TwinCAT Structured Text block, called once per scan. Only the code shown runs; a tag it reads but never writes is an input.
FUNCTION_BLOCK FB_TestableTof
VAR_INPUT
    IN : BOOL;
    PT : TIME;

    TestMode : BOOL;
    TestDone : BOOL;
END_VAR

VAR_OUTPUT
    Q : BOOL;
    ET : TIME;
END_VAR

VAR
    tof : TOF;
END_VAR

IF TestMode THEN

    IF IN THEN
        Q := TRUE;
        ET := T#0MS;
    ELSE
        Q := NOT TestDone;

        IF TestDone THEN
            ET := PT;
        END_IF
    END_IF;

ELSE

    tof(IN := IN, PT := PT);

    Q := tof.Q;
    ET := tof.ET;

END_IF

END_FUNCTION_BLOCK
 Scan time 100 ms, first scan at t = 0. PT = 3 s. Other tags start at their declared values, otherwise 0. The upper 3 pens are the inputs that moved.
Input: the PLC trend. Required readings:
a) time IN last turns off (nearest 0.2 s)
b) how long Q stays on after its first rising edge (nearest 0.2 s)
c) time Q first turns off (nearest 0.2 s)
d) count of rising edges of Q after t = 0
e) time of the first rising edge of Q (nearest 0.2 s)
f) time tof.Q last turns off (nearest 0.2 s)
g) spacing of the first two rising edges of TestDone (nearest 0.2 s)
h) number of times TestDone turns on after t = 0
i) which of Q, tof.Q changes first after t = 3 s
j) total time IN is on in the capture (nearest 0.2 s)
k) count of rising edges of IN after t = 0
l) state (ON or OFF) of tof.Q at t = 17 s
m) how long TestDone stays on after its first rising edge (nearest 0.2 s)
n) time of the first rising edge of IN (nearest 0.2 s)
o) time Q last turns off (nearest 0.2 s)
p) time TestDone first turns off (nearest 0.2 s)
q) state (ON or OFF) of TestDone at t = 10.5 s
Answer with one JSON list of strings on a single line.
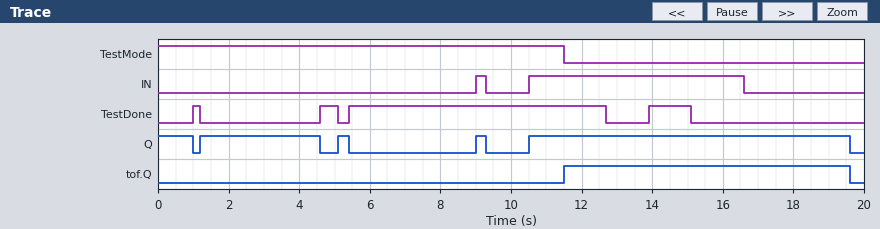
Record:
["16.6 s", "3.4 s", "1.0 s", "4", "1.2 s", "19.6 s", "3.6 s", "4", "Q", "6.4 s", "2", "ON", "0.2 s", "9.0 s", "19.6 s", "1.2 s", "ON"]
